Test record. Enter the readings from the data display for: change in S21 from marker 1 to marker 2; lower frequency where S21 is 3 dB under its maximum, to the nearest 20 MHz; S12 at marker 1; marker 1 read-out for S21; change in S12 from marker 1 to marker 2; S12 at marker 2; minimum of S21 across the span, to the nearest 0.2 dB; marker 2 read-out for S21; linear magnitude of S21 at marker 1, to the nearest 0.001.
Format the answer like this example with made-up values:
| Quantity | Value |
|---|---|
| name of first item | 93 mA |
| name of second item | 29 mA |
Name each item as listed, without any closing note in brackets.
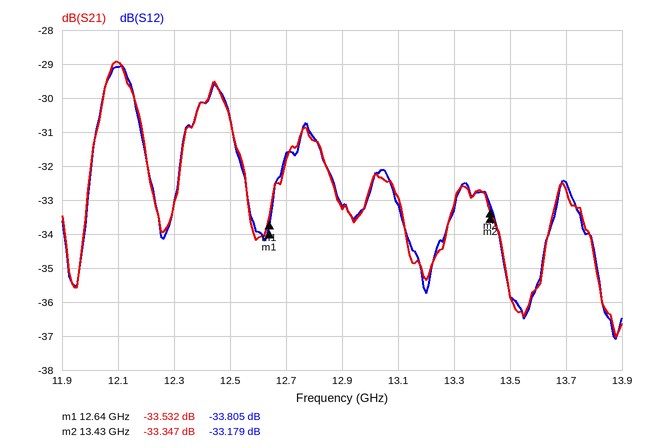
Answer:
| Quantity | Value |
|---|---|
| change in S21 from marker 1 to marker 2 | 0.185 dB |
| lower frequency where S21 is 3 dB under its maximum, to the nearest 20 MHz | 12.00 GHz |
| S12 at marker 1 | -33.805 dB |
| marker 1 read-out for S21 | -33.532 dB |
| change in S12 from marker 1 to marker 2 | 0.626 dB |
| S12 at marker 2 | -33.179 dB |
| minimum of S21 across the span, to the nearest 0.2 dB | -37.0 dB |
| marker 2 read-out for S21 | -33.347 dB |
| linear magnitude of S21 at marker 1, to the nearest 0.001 | 0.021 |
